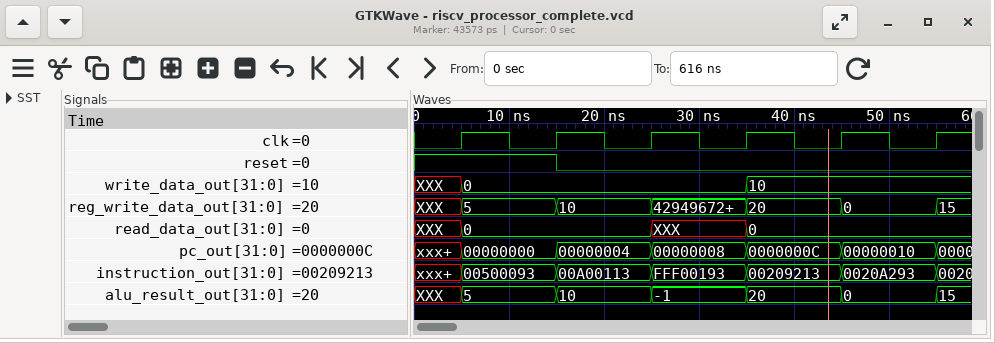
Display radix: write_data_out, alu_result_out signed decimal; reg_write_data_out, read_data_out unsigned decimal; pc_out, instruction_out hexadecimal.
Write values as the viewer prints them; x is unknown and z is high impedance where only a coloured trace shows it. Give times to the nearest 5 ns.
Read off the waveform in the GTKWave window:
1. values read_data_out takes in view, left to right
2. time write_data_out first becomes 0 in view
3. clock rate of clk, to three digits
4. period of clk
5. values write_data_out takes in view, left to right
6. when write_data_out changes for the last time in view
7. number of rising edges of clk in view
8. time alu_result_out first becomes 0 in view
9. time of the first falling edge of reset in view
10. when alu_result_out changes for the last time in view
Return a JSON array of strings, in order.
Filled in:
["XXX, 0, XXX, 0", "5 ns", "100 MHz", "10 ns", "XXX, 0, 10", "35 ns", "6", "45 ns", "15 ns", "55 ns"]
